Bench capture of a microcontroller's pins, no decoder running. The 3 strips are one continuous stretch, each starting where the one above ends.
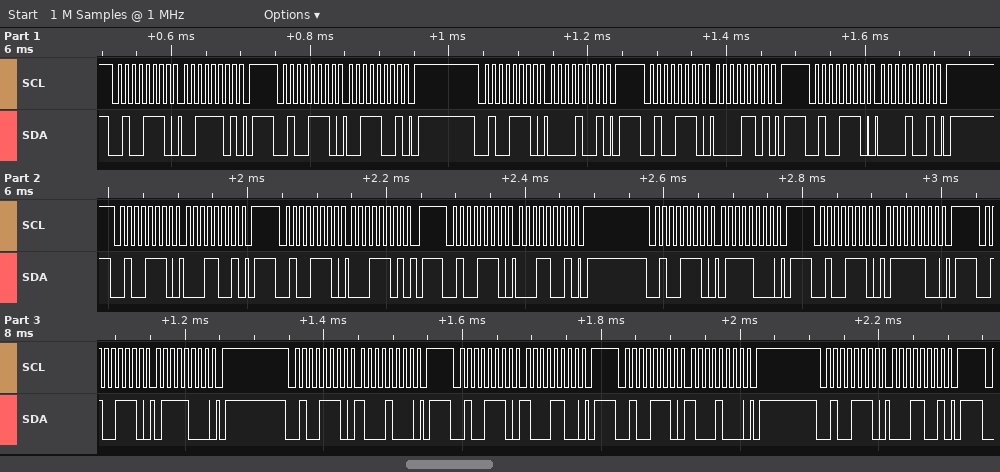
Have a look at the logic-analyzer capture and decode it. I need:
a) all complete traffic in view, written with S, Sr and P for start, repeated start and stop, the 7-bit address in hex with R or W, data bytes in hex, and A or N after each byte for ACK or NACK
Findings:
S 27W A 3D A P S 27W A 39 A P S 27W A 09 A P S 27W A 0D A P S 27W A 09 A P S 27W A 19 A P S 27W A 1D A P S 27W A 19 A P S 27W A 78 A P S 27W A 7C A P S 27W A 78 A P S 27W A 88 A P S 27W A 8C A P S 27W A 88 A P S 27W A 19 A P
